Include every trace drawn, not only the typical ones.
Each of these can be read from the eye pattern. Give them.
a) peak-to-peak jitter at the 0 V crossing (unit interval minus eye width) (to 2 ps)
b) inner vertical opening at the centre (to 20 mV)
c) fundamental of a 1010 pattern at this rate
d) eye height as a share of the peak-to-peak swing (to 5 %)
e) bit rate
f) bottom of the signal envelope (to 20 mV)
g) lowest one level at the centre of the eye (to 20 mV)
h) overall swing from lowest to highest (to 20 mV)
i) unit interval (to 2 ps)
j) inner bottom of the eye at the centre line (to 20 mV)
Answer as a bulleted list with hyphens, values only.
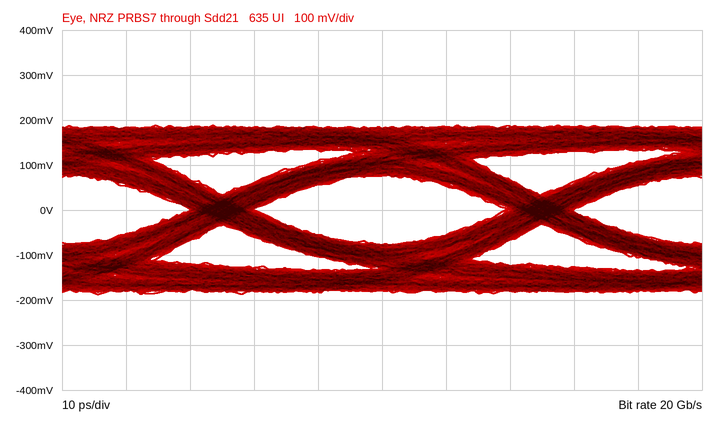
- 10 ps
- 160 mV
- 10 GHz
- 40 %
- 20 Gb/s
- -180 mV
- 80 mV
- 380 mV
- 50 ps
- -80 mV
